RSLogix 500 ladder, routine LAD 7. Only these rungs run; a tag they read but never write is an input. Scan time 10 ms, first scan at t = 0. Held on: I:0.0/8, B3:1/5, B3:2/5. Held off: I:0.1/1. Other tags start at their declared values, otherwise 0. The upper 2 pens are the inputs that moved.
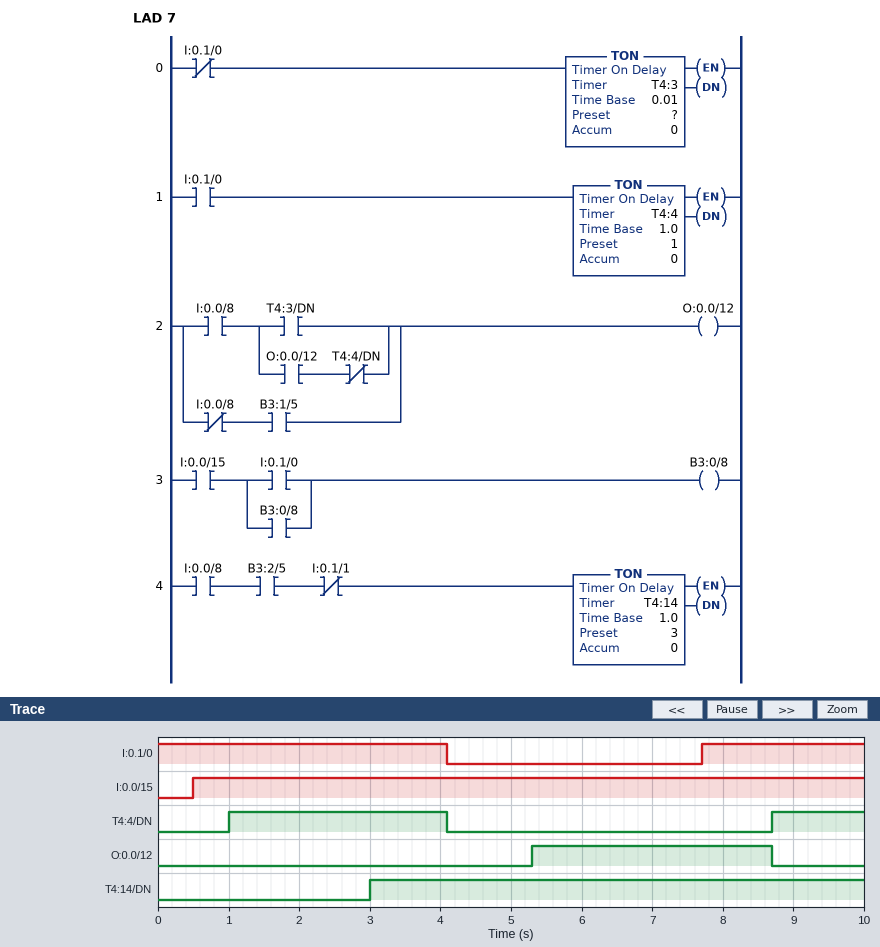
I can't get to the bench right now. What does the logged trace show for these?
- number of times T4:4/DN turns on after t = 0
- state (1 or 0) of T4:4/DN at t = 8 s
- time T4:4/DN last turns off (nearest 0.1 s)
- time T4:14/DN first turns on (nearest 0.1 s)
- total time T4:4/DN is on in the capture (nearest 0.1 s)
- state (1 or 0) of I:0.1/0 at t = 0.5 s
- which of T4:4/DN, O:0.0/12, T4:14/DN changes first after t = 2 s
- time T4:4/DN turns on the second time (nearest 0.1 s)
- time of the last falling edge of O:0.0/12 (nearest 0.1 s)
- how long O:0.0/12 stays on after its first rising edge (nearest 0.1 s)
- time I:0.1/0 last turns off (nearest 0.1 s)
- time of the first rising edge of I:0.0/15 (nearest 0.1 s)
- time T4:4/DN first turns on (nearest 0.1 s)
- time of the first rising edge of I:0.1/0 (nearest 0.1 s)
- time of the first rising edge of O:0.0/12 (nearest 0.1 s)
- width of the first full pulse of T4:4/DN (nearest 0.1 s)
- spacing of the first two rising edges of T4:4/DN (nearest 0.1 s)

2
0
4.1 s
3.0 s
4.4 s
1
T4:14/DN
8.7 s
8.7 s
3.4 s
4.1 s
0.5 s
1.0 s
7.7 s
5.3 s
3.1 s
7.7 s
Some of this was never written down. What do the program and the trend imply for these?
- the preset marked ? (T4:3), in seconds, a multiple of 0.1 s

1.2 s
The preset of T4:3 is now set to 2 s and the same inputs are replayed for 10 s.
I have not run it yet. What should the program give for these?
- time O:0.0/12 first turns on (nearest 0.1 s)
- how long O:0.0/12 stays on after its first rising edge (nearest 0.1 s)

6.1 s
2.6 s
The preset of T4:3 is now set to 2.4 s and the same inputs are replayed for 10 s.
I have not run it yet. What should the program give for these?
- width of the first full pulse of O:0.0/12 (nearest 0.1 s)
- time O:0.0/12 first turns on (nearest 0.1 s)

2.2 s
6.5 s
